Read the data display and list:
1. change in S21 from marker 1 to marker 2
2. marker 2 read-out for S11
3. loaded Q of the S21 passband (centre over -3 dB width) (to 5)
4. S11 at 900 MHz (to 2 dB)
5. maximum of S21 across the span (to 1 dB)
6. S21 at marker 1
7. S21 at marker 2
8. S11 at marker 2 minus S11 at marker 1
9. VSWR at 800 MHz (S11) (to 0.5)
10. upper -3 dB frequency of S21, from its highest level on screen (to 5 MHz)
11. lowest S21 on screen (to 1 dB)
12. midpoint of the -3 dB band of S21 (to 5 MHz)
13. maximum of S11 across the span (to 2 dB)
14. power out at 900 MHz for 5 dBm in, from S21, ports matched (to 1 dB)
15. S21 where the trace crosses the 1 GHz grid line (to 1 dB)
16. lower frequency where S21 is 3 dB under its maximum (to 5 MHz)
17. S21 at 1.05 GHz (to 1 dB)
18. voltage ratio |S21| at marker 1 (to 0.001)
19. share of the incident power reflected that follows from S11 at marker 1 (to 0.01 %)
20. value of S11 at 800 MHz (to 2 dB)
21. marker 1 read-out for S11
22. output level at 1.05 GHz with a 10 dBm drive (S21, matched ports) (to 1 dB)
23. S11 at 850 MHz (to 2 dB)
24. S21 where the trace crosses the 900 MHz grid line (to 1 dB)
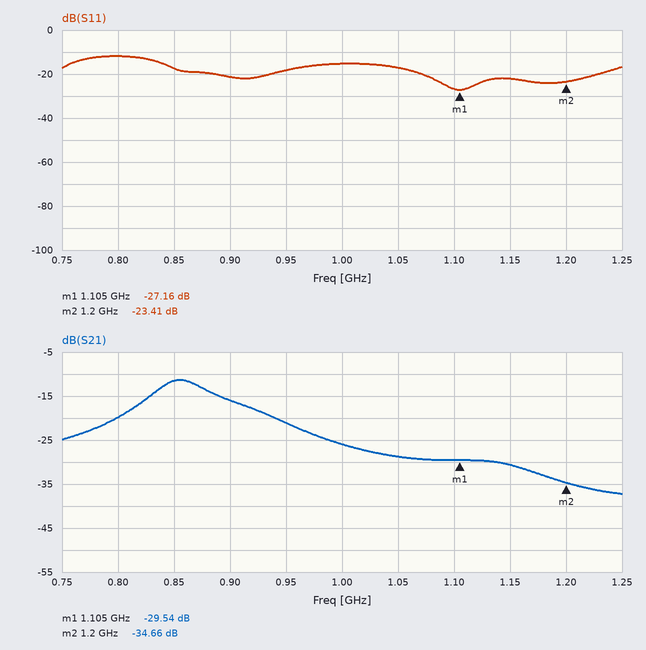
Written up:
-5.12 dB
-23.41 dB
15
-22 dB
-11 dB
-29.54 dB
-34.66 dB
3.75 dB
1.5
885 MHz
-37 dB
860 MHz
-12 dB
-11 dBm
-26 dB
830 MHz
-29 dB
0.033
0.19 %
-12 dB
-27.16 dB
-19 dBm
-18 dB
-16 dB
